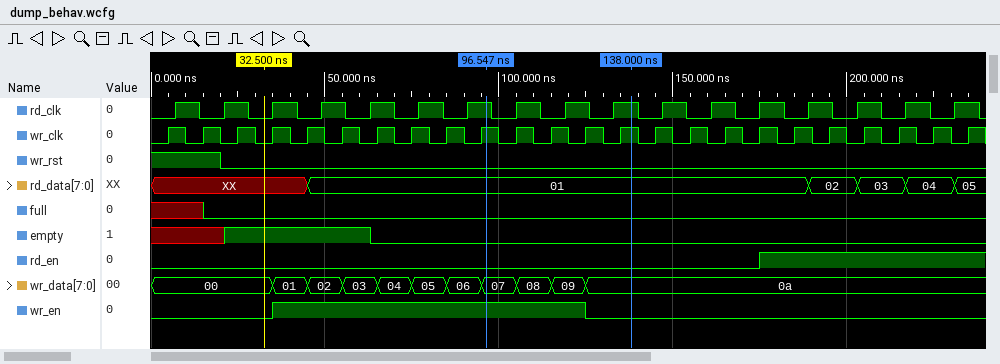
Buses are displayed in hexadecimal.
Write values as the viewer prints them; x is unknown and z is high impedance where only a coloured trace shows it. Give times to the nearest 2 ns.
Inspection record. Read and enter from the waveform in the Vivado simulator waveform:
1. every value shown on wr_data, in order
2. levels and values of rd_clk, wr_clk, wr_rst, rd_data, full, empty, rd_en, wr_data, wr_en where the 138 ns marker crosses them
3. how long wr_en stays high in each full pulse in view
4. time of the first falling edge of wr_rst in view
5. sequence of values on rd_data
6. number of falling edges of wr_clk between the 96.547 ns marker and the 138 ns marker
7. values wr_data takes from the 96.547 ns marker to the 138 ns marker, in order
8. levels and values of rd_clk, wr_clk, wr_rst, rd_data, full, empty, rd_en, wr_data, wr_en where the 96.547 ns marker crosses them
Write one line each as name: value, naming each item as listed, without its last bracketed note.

every value shown on wr_data, in order: 00, 01, 02, 03, 04, 05, 06, 07, 08, 09, 0a
levels and values of rd_clk, wr_clk, wr_rst, rd_data, full, empty, rd_en, wr_data, wr_en where the 138 ns marker crosses them: rd_clk=1, wr_clk=1, wr_rst=0, rd_data=01, full=0, empty=0, rd_en=0, wr_data=0a, wr_en=0
how long wr_en stays high in each full pulse in view: 90 ns
time of the first falling edge of wr_rst in view: 20 ns
sequence of values on rd_data: XX, 01, 02, 03, 04, 05
number of falling edges of wr_clk between the 96.547 ns marker and the 138 ns marker: 4
values wr_data takes from the 96.547 ns marker to the 138 ns marker, in order: 07, 08, 09, 0a
levels and values of rd_clk, wr_clk, wr_rst, rd_data, full, empty, rd_en, wr_data, wr_en where the 96.547 ns marker crosses them: rd_clk=1, wr_clk=1, wr_rst=0, rd_data=01, full=0, empty=0, rd_en=0, wr_data=07, wr_en=1
